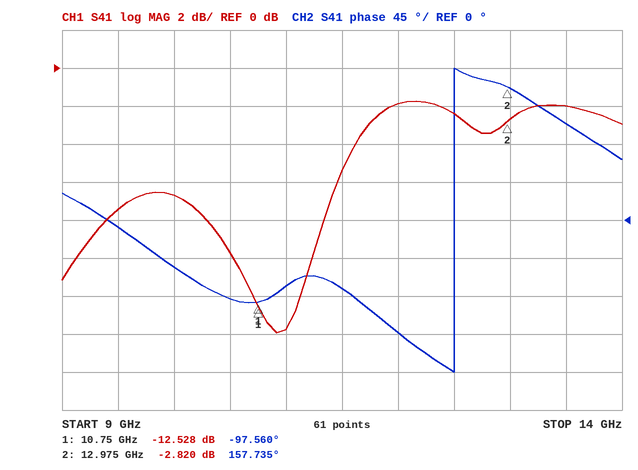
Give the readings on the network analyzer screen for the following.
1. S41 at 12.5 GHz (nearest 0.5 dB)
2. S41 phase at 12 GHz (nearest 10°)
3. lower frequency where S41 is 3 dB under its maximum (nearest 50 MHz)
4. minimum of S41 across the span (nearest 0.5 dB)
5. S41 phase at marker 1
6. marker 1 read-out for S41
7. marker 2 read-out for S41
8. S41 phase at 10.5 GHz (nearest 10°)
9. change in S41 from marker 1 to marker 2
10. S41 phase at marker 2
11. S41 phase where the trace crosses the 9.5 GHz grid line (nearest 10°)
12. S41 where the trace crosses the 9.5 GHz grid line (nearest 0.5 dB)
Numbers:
-2.5 dB
-130°
11.55 GHz
-14.0 dB
-97.560°
-12.528 dB
-2.820 dB
-90°
9.708 dB
157.735°
-10°
-7.5 dB
